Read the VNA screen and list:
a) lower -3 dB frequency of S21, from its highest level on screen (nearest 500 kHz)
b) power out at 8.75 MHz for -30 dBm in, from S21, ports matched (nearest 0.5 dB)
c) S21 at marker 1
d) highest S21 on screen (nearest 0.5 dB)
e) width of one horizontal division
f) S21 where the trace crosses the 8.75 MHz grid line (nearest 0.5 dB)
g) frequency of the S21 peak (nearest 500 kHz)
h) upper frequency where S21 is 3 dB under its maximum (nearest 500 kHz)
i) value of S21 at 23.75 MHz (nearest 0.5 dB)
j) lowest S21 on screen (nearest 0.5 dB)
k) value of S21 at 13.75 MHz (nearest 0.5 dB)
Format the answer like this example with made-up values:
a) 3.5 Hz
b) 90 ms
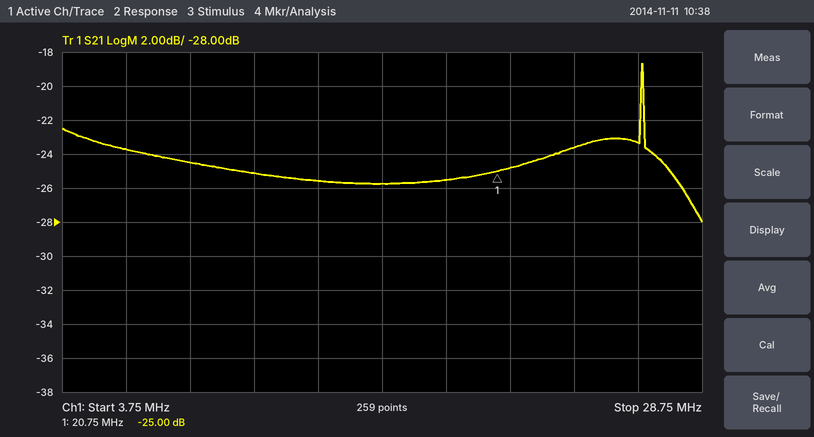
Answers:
a) 26.5 MHz
b) -54.5 dBm
c) -25.00 dB
d) -18.5 dB
e) 2.5 MHz
f) -24.5 dB
g) 26.5 MHz
h) 26.5 MHz
i) -23.5 dB
j) -28.0 dB
k) -25.5 dB
